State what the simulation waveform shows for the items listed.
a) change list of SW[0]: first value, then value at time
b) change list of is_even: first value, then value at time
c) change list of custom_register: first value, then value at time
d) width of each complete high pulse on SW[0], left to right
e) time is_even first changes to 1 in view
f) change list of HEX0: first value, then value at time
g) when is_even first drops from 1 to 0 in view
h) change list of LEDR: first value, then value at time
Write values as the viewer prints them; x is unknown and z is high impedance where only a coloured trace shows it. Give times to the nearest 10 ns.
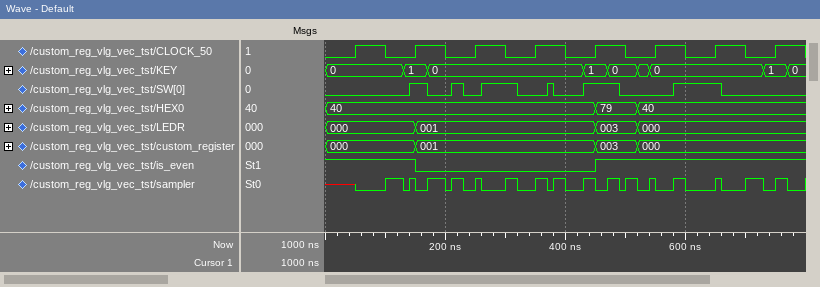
0, 1 at 140 ns, 0 at 170 ns, 1 at 210 ns, 0 at 230 ns, 1 at 260 ns, 0 at 320 ns, 1 at 370 ns, 0 at 380 ns, 1 at 430 ns, 0 at 490 ns, 1 at 580 ns, 0 at 660 ns
1, 0 at 150 ns, 1 at 450 ns
000, 001 at 150 ns, 003 at 450 ns, 000 at 520 ns
30 ns, 20 ns, 60 ns, 10 ns, 60 ns, 80 ns
450 ns
40, 79 at 450 ns, 40 at 520 ns
150 ns
000, 001 at 150 ns, 003 at 450 ns, 000 at 520 ns
